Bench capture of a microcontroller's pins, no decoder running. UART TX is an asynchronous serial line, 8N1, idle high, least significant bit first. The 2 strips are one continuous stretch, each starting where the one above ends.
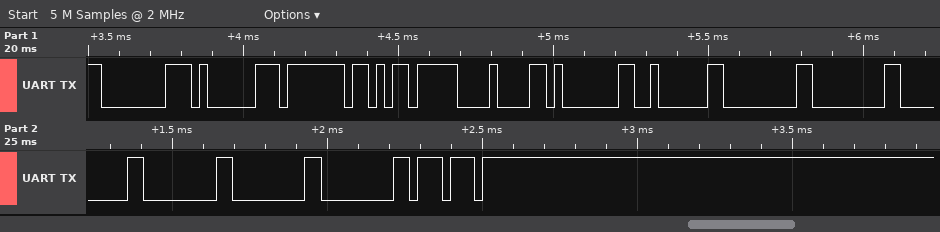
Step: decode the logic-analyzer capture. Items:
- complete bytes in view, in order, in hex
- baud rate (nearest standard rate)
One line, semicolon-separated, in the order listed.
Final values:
0x80 0x81 0x7F 0xED 0x08 0x01 0x02 0x00 0x00 0x00 0x00 0x00 0x00 0x77; 38400 baud
